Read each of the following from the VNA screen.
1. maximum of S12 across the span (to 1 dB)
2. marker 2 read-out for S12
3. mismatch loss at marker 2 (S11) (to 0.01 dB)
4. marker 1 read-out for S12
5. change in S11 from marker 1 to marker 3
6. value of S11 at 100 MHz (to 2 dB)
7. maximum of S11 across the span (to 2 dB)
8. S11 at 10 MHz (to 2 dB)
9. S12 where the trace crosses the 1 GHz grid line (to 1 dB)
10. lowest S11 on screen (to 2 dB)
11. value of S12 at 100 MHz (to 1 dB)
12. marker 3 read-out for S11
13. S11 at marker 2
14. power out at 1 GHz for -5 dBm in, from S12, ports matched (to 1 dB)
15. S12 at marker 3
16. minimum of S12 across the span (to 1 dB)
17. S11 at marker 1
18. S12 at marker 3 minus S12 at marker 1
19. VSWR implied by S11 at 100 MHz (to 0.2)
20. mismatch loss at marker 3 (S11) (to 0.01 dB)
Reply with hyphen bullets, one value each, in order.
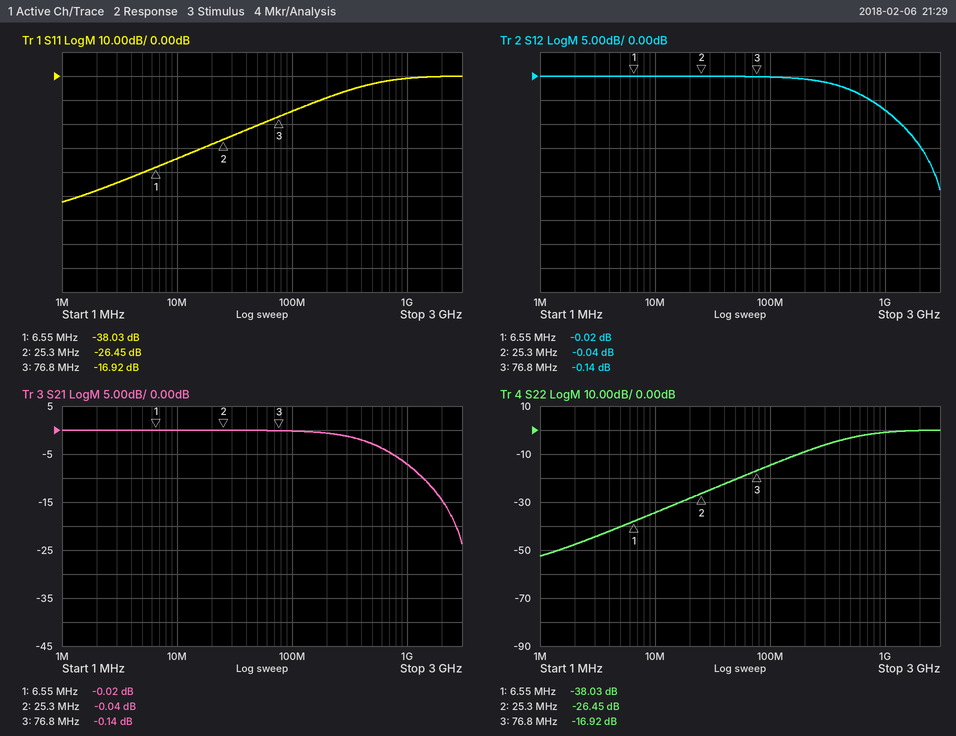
- 0 dB
- -0.04 dB
- 0.01 dB
- -0.02 dB
- 21.11 dB
- -14 dB
- 0 dB
- -34 dB
- -7 dB
- -52 dB
- 0 dB
- -16.92 dB
- -26.45 dB
- -12 dBm
- -0.14 dB
- -24 dB
- -38.03 dB
- -0.12 dB
- 1.4
- 0.09 dB
